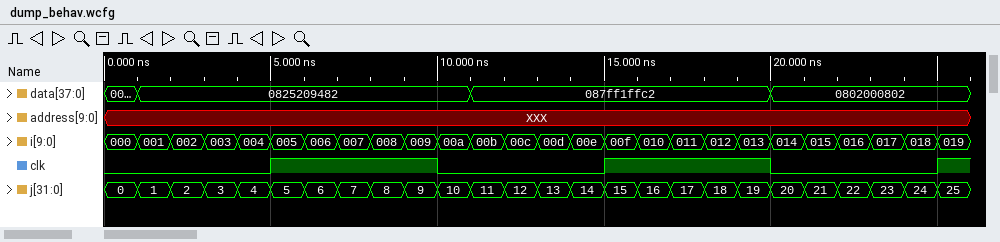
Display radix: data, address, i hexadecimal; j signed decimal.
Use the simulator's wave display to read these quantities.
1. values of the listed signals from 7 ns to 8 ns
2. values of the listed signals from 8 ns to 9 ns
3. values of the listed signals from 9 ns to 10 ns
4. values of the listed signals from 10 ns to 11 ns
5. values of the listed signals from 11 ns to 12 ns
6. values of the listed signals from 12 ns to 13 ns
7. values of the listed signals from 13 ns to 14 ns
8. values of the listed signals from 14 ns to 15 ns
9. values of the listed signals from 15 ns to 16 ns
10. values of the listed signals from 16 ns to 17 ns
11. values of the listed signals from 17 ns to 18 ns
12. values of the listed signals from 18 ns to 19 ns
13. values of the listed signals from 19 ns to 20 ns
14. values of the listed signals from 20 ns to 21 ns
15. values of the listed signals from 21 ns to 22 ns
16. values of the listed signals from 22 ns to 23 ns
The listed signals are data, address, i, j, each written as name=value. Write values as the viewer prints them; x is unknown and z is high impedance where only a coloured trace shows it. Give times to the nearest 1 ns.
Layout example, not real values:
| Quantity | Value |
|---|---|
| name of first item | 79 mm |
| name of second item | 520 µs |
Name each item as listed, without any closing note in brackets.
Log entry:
| Quantity | Value |
|---|---|
| values of the listed signals from 7 ns to 8 ns | data=0825209482, address=XXX, i=007, j=7 |
| values of the listed signals from 8 ns to 9 ns | data=0825209482, address=XXX, i=008, j=8 |
| values of the listed signals from 9 ns to 10 ns | data=0825209482, address=XXX, i=009, j=9 |
| values of the listed signals from 10 ns to 11 ns | data=0825209482, address=XXX, i=00a, j=10 |
| values of the listed signals from 11 ns to 12 ns | data=087ff1ffc2, address=XXX, i=00b, j=11 |
| values of the listed signals from 12 ns to 13 ns | data=087ff1ffc2, address=XXX, i=00c, j=12 |
| values of the listed signals from 13 ns to 14 ns | data=087ff1ffc2, address=XXX, i=00d, j=13 |
| values of the listed signals from 14 ns to 15 ns | data=087ff1ffc2, address=XXX, i=00e, j=14 |
| values of the listed signals from 15 ns to 16 ns | data=087ff1ffc2, address=XXX, i=00f, j=15 |
| values of the listed signals from 16 ns to 17 ns | data=087ff1ffc2, address=XXX, i=010, j=16 |
| values of the listed signals from 17 ns to 18 ns | data=087ff1ffc2, address=XXX, i=011, j=17 |
| values of the listed signals from 18 ns to 19 ns | data=087ff1ffc2, address=XXX, i=012, j=18 |
| values of the listed signals from 19 ns to 20 ns | data=087ff1ffc2, address=XXX, i=013, j=19 |
| values of the listed signals from 20 ns to 21 ns | data=0802000802, address=XXX, i=014, j=20 |
| values of the listed signals from 21 ns to 22 ns | data=0802000802, address=XXX, i=015, j=21 |
| values of the listed signals from 22 ns to 23 ns | data=0802000802, address=XXX, i=016, j=22 |
